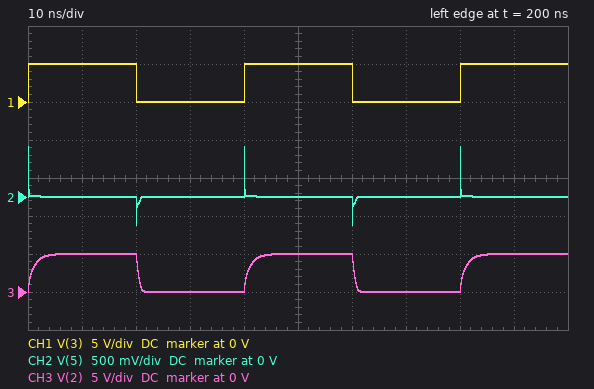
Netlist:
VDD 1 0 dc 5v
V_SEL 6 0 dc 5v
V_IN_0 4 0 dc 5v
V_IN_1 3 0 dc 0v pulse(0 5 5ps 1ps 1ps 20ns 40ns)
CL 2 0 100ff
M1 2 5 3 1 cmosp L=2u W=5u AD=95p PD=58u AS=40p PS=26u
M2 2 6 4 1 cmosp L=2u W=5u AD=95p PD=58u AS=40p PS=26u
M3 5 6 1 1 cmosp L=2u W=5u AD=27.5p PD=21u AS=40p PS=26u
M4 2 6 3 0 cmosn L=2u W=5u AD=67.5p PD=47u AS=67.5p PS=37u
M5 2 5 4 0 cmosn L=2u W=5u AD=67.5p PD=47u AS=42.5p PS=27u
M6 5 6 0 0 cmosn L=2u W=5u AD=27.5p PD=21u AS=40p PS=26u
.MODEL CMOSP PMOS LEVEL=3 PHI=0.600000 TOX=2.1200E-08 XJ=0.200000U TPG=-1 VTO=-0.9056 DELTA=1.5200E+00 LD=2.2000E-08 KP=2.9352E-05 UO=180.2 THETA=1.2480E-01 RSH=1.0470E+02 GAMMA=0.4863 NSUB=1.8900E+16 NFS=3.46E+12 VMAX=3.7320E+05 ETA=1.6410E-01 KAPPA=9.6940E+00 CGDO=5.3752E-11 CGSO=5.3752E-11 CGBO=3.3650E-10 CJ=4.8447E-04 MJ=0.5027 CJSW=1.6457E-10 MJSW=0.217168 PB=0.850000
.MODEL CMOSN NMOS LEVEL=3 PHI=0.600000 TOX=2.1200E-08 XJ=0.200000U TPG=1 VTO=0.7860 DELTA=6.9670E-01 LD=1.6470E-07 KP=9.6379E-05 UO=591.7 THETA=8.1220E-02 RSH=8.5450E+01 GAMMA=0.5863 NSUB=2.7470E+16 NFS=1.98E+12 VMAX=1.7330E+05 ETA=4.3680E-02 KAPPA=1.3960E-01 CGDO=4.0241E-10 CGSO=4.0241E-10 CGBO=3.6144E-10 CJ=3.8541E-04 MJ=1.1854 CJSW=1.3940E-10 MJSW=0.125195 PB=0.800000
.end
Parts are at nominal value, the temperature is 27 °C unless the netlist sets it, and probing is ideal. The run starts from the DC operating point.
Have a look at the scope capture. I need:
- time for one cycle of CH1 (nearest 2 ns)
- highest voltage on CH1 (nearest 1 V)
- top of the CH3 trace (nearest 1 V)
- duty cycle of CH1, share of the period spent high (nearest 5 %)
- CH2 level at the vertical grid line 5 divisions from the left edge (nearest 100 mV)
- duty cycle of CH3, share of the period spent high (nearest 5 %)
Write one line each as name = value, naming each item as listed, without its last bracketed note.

time for one cycle of CH1 = 40 ns
highest voltage on CH1 = 5 V
top of the CH3 trace = 5 V
duty cycle of CH1, share of the period spent high = 50 %
CH2 level at the vertical grid line 5 divisions from the left edge = 0 V
duty cycle of CH3, share of the period spent high = 50 %
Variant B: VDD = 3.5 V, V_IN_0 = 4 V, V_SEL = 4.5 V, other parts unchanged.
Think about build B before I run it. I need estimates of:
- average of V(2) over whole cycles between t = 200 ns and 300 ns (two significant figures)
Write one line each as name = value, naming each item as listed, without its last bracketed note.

average of V(2) over whole cycles between t = 200 ns and 300 ns = 2.0 V
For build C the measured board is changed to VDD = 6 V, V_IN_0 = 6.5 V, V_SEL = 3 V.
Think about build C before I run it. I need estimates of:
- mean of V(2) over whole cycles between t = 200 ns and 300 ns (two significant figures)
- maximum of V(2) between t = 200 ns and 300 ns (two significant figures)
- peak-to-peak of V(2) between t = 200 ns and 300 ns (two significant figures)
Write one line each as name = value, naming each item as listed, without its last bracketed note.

mean of V(2) over whole cycles between t = 200 ns and 300 ns = 3.0 V
maximum of V(2) between t = 200 ns and 300 ns = 5.6 V
peak-to-peak of V(2) between t = 200 ns and 300 ns = 5.2 V
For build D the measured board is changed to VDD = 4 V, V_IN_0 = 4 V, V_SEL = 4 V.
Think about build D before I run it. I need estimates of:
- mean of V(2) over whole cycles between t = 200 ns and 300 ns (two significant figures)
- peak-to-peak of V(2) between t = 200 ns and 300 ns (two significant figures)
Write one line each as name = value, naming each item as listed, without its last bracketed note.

mean of V(2) over whole cycles between t = 200 ns and 300 ns = 2.2 V
peak-to-peak of V(2) between t = 200 ns and 300 ns = 4.5 V
